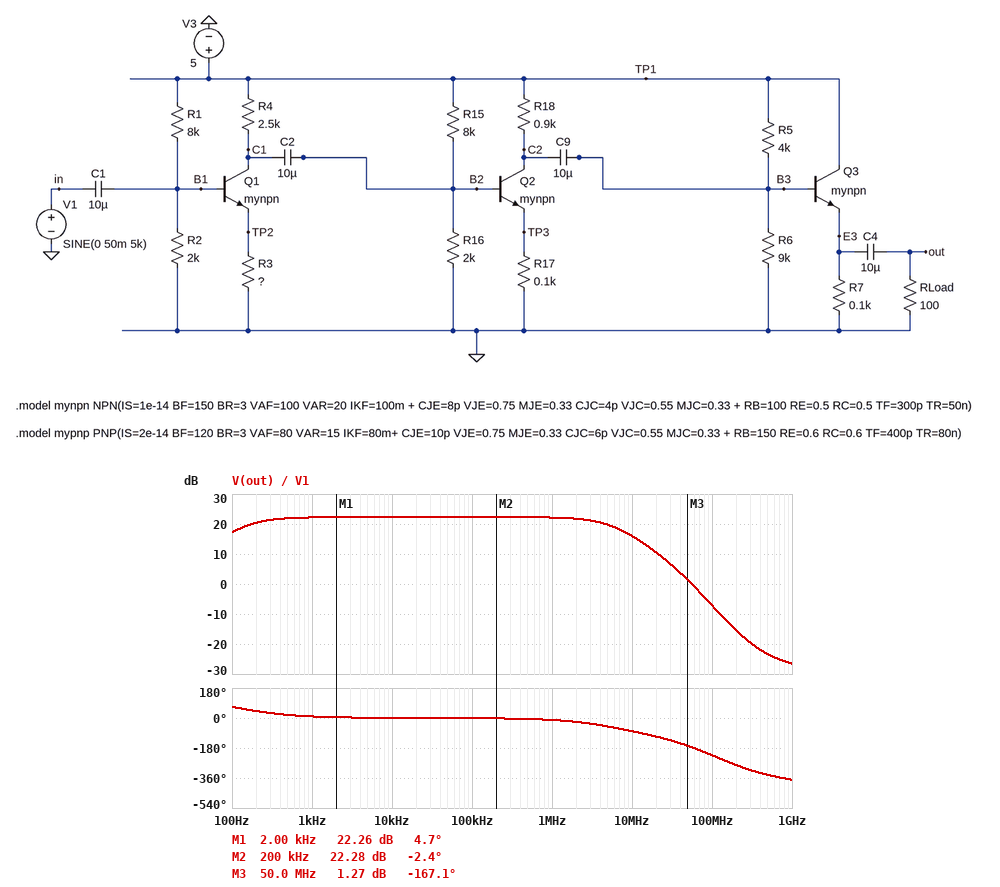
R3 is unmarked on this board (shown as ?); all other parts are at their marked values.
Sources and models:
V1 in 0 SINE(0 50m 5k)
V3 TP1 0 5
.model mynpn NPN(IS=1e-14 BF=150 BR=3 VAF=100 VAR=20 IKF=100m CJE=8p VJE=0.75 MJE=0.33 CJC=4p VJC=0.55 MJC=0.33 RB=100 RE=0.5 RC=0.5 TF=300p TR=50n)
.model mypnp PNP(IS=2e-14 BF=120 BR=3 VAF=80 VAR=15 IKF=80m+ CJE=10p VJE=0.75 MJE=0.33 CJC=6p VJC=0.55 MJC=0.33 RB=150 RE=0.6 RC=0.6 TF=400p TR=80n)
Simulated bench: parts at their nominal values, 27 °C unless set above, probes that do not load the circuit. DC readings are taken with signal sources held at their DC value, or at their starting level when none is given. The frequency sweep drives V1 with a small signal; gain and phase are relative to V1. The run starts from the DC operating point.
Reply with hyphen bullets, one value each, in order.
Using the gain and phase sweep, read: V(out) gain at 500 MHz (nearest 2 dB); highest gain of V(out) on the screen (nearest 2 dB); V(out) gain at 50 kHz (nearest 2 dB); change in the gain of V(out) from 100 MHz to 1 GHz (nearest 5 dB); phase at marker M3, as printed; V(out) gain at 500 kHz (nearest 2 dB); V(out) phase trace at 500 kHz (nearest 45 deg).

- -24 dB
- 22 dB
- 22 dB
- -20 dB
- -167.1 deg
- 22 dB
- 0 deg
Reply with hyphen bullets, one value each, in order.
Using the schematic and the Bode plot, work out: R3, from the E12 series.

- 330 Ω
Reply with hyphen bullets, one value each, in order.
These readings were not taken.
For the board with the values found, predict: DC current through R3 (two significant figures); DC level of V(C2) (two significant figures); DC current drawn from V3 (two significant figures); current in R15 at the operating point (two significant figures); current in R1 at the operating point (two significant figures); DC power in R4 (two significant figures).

- 1.0 mA
- 2.5 V
- 27 mA
- 500 µA
- 500 µA
- 2.5 mW
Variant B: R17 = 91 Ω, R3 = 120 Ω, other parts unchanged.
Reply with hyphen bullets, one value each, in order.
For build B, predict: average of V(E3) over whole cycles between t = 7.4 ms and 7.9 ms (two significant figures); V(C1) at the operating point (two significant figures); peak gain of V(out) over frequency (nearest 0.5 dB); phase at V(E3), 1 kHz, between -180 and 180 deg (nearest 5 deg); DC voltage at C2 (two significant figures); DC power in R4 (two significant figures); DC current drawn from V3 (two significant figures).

- 1.9 V
- 310 mV
- 16.5 dB
- 5 deg
- 2.3 V
- 8.8 mW
- 28 mA
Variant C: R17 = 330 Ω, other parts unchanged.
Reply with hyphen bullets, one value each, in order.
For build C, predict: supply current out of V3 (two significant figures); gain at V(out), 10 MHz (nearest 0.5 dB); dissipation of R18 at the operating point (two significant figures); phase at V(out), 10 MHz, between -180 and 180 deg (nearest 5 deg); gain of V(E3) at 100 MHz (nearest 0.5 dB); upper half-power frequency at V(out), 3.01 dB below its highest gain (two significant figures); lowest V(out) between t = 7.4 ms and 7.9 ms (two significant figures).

- 25 mA
- 9.5 dB
- 900 µW
- -65 deg
- -11.5 dB
- 10 MHz
- -210 mV
